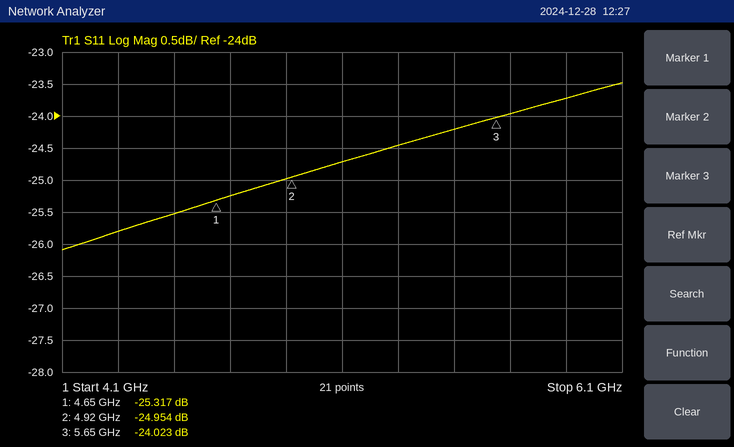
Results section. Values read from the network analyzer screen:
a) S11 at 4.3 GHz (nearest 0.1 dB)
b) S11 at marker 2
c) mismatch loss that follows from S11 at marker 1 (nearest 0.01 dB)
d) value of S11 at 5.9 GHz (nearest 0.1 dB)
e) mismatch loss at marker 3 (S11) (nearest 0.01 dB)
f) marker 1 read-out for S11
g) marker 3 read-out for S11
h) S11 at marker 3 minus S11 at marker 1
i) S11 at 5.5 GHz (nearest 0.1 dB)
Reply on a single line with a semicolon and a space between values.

-25.8 dB; -24.954 dB; 0.01 dB; -23.7 dB; 0.02 dB; -25.317 dB; -24.023 dB; 1.294 dB; -24.2 dB
